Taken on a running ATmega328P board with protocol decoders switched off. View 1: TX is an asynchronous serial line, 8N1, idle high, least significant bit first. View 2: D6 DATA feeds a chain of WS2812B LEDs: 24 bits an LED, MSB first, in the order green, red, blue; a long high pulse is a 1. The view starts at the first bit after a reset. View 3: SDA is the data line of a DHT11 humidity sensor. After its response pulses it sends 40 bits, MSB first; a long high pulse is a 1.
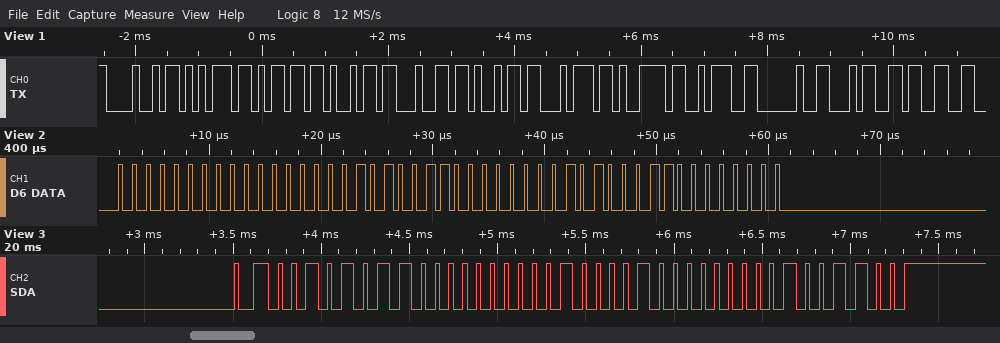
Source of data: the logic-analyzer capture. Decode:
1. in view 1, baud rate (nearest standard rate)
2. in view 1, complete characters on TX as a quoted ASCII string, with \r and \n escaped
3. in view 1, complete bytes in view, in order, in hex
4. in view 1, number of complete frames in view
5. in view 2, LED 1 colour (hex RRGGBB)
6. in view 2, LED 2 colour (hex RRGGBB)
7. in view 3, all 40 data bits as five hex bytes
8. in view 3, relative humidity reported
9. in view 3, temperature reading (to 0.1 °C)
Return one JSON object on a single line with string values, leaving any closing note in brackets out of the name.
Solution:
{"in view 1, baud rate": "9600 baud", "in view 1, complete characters on TX as a quoted ASCII string, with \\r and \\n escaped": "\"Humidity: 43\"", "in view 1, complete bytes in view, in order, in hex": "48 75 6D 69 64 69 74 79 3A 20 34 33", "in view 1, number of complete frames in view": "12", "in view 2, LED 1 colour": "#000053", "in view 2, LED 2 colour": "#A30000", "in view 3, all 40 data bits as five hex bytes": "2B 00 21 00 4C", "in view 3, relative humidity reported": "43 %", "in view 3, temperature reading": "33.0 °C"}
